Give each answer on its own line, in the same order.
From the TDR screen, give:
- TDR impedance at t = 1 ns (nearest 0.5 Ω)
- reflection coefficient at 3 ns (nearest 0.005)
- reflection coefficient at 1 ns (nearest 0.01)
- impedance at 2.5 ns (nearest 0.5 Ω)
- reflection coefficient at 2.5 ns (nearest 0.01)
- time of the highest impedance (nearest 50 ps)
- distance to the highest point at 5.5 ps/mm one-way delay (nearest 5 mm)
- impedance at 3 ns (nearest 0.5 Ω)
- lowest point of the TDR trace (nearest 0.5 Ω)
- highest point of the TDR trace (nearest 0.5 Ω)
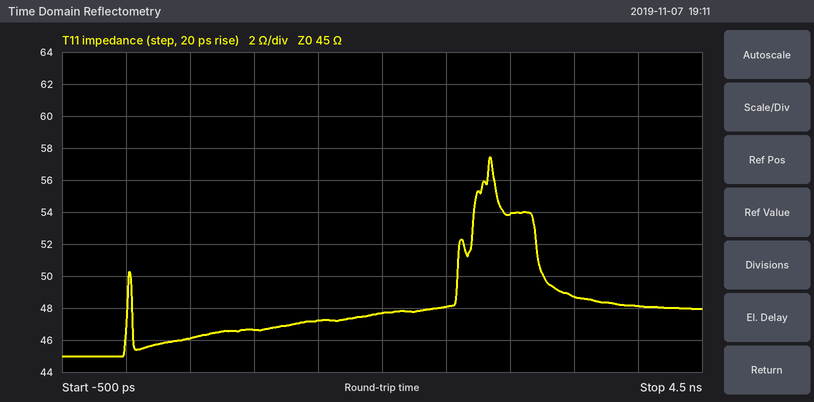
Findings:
46.5 Ω
+0.090
+0.02
48.0 Ω
+0.03
2.85 ns
260 mm
54.0 Ω
45.0 Ω
57.5 Ω
